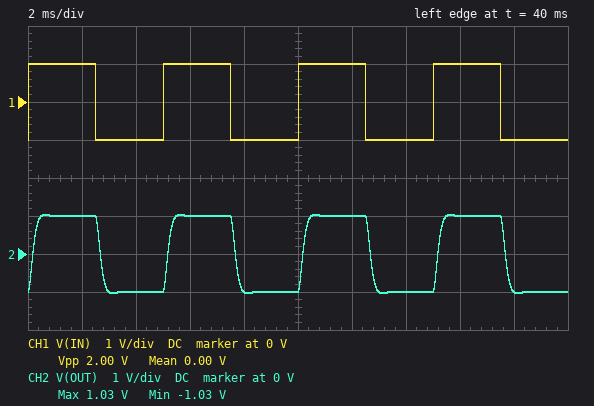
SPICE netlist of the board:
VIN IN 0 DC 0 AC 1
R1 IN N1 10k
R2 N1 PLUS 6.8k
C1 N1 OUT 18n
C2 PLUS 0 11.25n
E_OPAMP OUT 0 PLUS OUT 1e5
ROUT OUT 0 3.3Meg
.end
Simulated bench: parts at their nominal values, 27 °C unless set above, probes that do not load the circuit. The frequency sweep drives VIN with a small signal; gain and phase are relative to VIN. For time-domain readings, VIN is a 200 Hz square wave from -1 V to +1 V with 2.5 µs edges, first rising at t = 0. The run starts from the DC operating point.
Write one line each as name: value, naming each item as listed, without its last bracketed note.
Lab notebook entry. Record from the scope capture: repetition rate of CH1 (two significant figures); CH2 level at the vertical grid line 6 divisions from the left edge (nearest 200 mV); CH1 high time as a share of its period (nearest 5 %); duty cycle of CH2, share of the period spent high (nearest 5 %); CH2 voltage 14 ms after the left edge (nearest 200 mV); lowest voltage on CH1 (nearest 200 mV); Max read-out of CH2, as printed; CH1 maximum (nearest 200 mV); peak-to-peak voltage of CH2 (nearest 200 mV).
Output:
repetition rate of CH1: 200 Hz
CH2 level at the vertical grid line 6 divisions from the left edge: 1.0 V
CH1 high time as a share of its period: 50 %
duty cycle of CH2, share of the period spent high: 50 %
CH2 voltage 14 ms after the left edge: -1.0 V
lowest voltage on CH1: -1.0 V
Max read-out of CH2, as printed: 1.03 V
CH1 maximum: 1.0 V
peak-to-peak voltage of CH2: 2.0 V
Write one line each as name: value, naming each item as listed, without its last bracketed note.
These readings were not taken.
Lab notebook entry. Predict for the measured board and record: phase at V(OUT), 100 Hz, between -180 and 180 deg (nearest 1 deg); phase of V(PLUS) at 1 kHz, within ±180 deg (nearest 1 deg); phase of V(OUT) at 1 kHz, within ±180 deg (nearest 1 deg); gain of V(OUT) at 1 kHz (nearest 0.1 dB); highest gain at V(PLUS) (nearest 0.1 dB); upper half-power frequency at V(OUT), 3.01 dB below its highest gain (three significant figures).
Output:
phase at V(OUT), 100 Hz, between -180 and 180 deg: -7 deg
phase of V(PLUS) at 1 kHz, within ±180 deg: -69 deg
phase of V(OUT) at 1 kHz, within ±180 deg: -69 deg
gain of V(OUT) at 1 kHz: -2.1 dB
highest gain at V(PLUS): 0 dB
upper half-power frequency at V(OUT), 3.01 dB below its highest gain: 1.17 kHz
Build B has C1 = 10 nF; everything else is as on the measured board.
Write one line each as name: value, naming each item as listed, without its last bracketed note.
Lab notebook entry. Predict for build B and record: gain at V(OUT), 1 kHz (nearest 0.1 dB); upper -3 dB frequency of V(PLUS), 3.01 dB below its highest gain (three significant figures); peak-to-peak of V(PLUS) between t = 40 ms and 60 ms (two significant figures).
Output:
gain at V(OUT), 1 kHz: -2.8 dB
upper -3 dB frequency of V(PLUS), 3.01 dB below its highest gain: 1.05 kHz
peak-to-peak of V(PLUS) between t = 40 ms and 60 ms: 2.0 V
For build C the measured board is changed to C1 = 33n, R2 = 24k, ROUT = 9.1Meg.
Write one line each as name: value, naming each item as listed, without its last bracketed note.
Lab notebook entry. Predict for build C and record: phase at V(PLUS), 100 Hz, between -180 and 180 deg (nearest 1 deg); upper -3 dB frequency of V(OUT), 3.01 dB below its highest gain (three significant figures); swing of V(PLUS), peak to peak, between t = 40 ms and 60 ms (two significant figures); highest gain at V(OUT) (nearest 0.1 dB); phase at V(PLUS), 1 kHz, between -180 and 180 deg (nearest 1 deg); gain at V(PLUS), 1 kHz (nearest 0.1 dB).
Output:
phase at V(PLUS), 100 Hz, between -180 and 180 deg: -14 deg
upper -3 dB frequency of V(OUT), 3.01 dB below its highest gain: 575 Hz
swing of V(PLUS), peak to peak, between t = 40 ms and 60 ms: 2.3 V
highest gain at V(OUT): 0.1 dB
phase at V(PLUS), 1 kHz, between -180 and 180 deg: -136 deg
gain at V(PLUS), 1 kHz: -10.8 dB
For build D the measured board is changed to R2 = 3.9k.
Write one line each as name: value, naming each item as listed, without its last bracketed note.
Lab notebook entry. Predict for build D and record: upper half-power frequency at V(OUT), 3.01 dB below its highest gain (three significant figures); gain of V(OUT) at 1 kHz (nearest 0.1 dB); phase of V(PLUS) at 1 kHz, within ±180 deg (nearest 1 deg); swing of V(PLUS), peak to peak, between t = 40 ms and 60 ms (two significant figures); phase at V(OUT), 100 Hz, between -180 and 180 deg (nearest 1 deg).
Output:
upper half-power frequency at V(OUT), 3.01 dB below its highest gain: 1.38 kHz
gain of V(OUT) at 1 kHz: -1.6 dB
phase of V(PLUS) at 1 kHz, within ±180 deg: -55 deg
swing of V(PLUS), peak to peak, between t = 40 ms and 60 ms: 2.0 V
phase at V(OUT), 100 Hz, between -180 and 180 deg: -6 deg
